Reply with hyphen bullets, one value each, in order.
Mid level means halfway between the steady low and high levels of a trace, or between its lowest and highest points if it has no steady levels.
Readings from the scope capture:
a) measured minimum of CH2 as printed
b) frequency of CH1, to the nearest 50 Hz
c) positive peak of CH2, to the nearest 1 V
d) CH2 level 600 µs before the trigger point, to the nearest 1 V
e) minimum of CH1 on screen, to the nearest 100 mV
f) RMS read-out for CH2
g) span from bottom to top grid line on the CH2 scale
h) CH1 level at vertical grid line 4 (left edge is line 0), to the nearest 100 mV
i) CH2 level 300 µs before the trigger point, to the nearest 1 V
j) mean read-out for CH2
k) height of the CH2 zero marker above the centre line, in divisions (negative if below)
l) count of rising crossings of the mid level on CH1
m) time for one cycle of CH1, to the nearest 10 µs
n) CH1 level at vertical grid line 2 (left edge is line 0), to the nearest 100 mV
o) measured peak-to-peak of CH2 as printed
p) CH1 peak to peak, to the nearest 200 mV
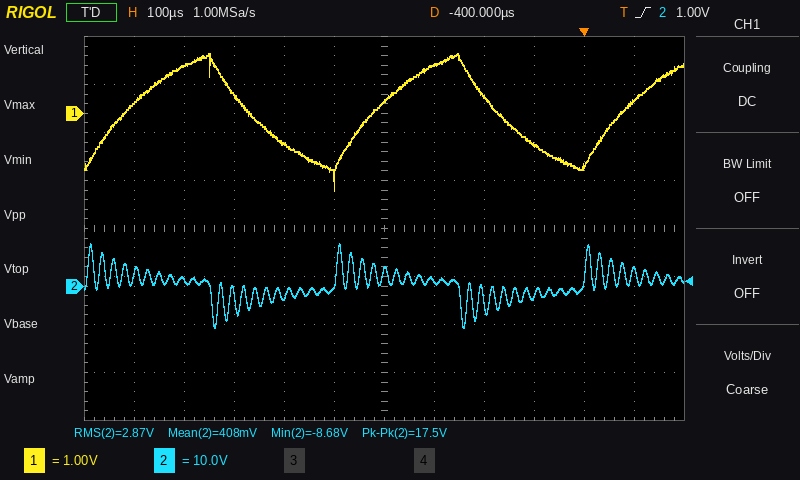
- -8.68 V
- 2.00 kHz
- 9 V
- -2 V
- -1.6 V
- 2.87 V
- 80 V
- -600 mV
- 1 V
- 408 mV
- -1.2 div
- 3
- 500 µs
- 1.0 V
- 17.5 V
- 2.8 V
